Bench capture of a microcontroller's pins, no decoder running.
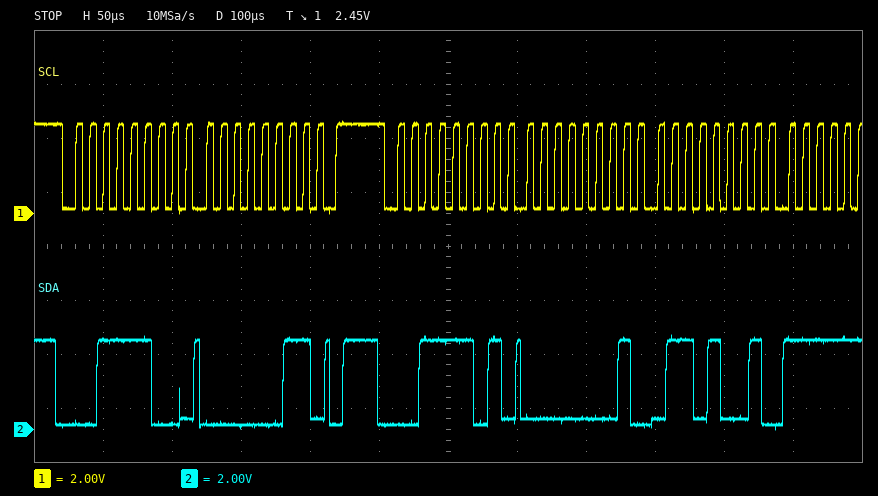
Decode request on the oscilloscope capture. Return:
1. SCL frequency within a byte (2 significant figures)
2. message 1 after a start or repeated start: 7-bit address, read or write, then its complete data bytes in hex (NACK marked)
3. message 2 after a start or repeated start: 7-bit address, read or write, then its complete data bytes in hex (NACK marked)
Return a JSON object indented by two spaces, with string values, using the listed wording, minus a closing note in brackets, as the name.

{
  "SCL frequency within a byte": "100 kHz",
  "message 1 after a start or repeated start: 7-bit address, read or write, then its complete data bytes in hex": "0x1E write: 03",
  "message 2 after a start or repeated start: 7-bit address, read or write, then its complete data bytes in hex": "0x1E read: 01 69"
}
